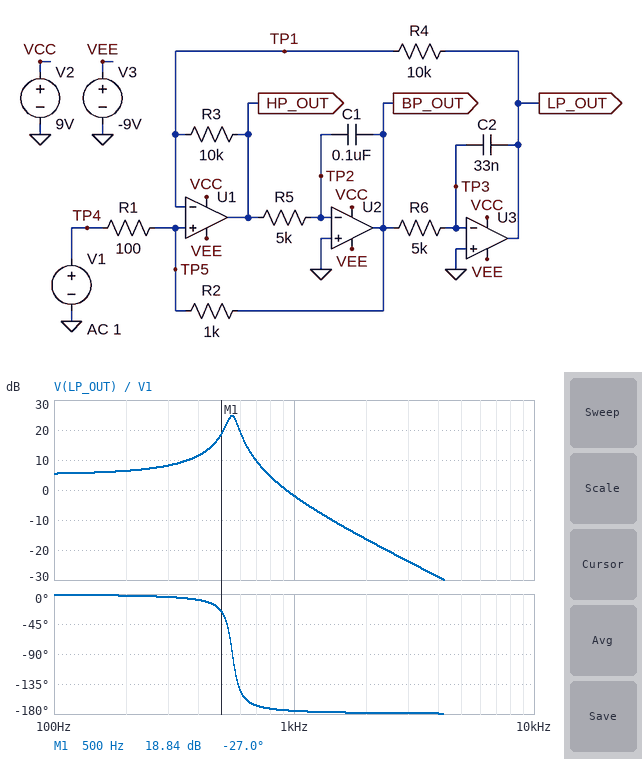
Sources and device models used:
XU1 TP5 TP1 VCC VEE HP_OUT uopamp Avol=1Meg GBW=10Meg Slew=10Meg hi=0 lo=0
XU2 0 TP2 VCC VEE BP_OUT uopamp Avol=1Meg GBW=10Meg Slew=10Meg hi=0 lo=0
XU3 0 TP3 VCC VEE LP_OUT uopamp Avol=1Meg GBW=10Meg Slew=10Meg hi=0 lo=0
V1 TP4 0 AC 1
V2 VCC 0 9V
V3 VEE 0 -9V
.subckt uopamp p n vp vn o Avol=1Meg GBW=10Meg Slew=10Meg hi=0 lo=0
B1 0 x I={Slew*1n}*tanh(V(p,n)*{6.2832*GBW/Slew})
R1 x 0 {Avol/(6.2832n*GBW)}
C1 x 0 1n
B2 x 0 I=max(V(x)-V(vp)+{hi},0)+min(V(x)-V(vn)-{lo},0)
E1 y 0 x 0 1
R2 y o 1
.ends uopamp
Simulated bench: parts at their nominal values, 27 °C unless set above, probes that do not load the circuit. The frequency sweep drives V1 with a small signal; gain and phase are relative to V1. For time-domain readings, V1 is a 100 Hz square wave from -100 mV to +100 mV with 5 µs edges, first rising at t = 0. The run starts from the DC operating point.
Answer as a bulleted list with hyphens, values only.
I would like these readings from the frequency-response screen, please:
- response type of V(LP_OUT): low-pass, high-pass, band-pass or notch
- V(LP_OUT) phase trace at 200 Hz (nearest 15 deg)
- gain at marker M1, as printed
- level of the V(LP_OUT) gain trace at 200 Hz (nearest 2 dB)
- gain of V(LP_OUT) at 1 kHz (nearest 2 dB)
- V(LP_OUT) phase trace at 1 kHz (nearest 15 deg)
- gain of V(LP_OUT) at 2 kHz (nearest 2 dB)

- low-pass
- 0 deg
- 18.84 dB
- 6 dB
- -2 dB
- -180 deg
- -16 dB
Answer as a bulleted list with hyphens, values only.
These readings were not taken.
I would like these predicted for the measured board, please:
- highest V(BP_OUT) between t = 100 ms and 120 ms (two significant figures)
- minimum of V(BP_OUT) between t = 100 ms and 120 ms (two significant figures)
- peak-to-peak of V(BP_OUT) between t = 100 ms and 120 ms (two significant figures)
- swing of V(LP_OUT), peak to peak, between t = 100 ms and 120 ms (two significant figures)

- 180 mV
- -180 mV
- 350 mV
- 930 mV
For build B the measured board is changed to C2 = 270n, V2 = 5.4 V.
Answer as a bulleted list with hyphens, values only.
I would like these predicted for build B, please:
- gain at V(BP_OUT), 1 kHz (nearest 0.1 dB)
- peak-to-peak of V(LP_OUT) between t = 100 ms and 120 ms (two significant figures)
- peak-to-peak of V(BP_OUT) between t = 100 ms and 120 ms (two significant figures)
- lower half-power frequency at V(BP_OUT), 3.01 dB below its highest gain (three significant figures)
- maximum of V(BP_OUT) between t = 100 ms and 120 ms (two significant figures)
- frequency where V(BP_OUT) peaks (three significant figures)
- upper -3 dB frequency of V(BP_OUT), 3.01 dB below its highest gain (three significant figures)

- -4.4 dB
- 690 mV
- 700 mV
- 167 Hz
- 350 mV
- 194 Hz
- 225 Hz
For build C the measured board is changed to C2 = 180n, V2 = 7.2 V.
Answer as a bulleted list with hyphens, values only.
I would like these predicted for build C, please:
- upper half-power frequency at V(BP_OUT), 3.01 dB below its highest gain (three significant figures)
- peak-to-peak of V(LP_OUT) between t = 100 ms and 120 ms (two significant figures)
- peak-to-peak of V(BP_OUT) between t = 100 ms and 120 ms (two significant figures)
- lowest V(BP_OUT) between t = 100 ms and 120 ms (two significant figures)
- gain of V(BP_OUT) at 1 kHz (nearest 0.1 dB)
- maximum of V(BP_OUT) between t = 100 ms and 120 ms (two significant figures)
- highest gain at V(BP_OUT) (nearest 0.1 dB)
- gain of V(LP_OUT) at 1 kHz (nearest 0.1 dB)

- 268 Hz
- 750 mV
- 640 mV
- -320 mV
- -4.3 dB
- 320 mV
- 20.0 dB
- -19.3 dB
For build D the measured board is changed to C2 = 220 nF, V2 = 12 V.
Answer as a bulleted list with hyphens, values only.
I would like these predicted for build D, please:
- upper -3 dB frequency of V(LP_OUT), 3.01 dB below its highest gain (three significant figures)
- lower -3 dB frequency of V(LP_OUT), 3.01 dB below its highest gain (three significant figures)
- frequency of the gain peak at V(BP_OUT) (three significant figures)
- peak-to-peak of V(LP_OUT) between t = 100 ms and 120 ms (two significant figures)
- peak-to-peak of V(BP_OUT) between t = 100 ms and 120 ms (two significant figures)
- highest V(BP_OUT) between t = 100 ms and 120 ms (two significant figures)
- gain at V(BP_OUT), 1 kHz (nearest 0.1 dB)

- 238 Hz
- 179 Hz
- 215 Hz
- 700 mV
- 630 mV
- 320 mV
- -4.4 dB
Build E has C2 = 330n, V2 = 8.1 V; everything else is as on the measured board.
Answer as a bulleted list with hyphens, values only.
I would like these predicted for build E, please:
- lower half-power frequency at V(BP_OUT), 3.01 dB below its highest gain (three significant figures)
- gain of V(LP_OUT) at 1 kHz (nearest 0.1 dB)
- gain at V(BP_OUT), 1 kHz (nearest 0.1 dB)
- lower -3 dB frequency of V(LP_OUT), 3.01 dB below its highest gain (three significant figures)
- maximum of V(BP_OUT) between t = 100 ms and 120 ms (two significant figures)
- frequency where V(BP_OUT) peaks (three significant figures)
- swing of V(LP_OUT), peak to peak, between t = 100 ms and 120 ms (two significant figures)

- 149 Hz
- -24.8 dB
- -4.5 dB
- 138 Hz
- 420 mV
- 175 Hz
- 710 mV
